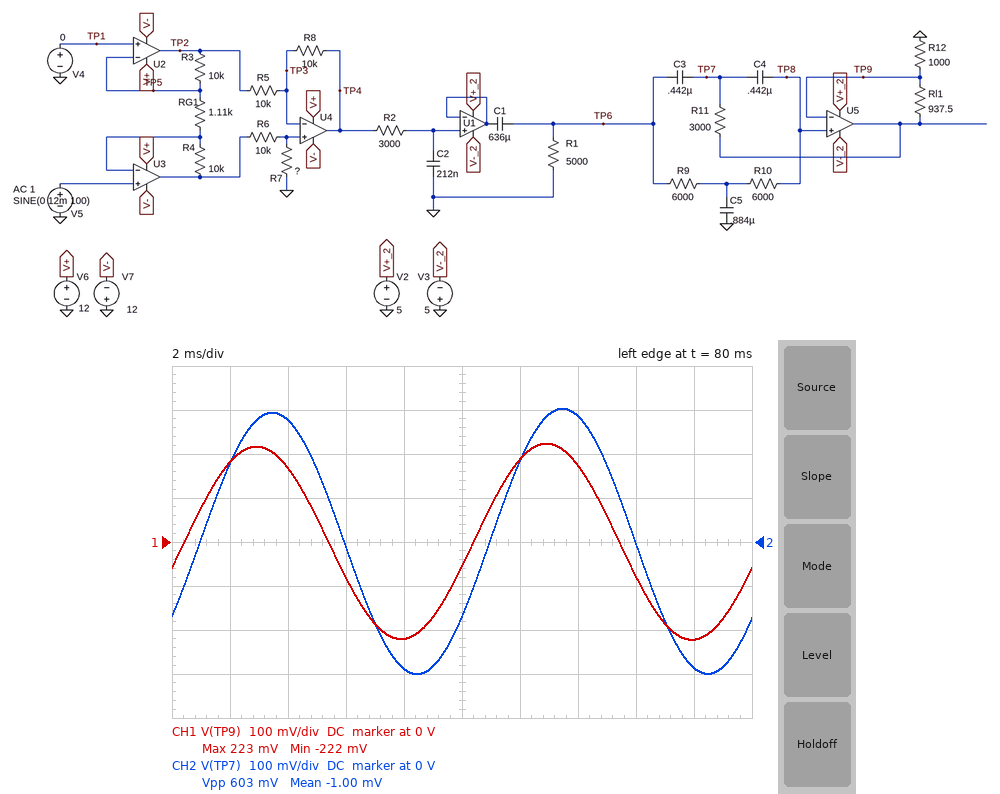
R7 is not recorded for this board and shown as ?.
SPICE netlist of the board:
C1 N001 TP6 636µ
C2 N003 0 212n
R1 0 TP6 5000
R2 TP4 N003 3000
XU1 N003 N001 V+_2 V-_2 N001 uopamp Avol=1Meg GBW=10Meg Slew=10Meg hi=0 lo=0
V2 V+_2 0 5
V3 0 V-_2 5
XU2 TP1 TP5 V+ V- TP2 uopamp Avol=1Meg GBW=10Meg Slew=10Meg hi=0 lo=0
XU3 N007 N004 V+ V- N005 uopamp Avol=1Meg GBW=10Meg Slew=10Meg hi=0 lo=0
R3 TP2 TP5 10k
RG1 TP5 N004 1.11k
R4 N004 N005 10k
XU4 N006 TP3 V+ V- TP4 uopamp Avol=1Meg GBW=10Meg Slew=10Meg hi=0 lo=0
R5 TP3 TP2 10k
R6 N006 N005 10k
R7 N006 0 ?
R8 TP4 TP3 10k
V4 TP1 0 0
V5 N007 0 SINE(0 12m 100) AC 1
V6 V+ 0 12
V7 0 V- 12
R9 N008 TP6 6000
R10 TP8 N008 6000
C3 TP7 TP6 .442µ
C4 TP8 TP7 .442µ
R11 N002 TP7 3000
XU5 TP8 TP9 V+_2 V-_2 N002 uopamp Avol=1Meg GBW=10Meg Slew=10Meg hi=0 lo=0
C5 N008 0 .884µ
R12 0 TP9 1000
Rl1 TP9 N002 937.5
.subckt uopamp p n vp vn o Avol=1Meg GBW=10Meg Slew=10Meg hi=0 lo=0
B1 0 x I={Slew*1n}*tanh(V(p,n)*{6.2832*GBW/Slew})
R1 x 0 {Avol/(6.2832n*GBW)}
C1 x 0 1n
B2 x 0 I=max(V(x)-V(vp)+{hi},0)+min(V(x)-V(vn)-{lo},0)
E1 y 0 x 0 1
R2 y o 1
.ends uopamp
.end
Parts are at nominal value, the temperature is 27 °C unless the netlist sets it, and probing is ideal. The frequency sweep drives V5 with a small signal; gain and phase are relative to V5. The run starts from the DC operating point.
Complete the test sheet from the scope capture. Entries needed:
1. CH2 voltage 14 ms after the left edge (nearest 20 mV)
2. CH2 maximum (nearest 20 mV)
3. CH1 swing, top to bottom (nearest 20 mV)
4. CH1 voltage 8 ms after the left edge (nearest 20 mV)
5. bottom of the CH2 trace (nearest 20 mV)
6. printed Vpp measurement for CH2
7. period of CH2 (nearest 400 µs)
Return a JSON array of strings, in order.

["280 mV", "300 mV", "440 mV", "-220 mV", "-300 mV", "603 mV", "10.0 ms"]
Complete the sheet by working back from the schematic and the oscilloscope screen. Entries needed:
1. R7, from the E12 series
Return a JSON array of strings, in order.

["12 kΩ"]
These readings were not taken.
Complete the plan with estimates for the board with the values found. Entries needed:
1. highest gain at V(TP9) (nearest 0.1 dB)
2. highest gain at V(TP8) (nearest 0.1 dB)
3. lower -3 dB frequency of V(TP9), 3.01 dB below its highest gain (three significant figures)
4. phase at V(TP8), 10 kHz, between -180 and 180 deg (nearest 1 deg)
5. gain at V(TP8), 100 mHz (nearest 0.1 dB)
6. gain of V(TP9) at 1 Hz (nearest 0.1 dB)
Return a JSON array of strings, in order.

["26.0 dB", "26.0 dB", "50.0 mHz", "-90 deg", "25.0 dB", "26.0 dB"]
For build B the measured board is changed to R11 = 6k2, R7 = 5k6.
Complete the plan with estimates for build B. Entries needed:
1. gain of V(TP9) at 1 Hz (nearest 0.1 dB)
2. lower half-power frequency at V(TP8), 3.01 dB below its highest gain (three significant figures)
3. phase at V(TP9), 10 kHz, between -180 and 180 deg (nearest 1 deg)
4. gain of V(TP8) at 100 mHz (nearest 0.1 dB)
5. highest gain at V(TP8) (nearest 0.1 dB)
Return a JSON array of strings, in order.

["24.2 dB", "78.4 mHz", "-90 deg", "23.2 dB", "25.7 dB"]
